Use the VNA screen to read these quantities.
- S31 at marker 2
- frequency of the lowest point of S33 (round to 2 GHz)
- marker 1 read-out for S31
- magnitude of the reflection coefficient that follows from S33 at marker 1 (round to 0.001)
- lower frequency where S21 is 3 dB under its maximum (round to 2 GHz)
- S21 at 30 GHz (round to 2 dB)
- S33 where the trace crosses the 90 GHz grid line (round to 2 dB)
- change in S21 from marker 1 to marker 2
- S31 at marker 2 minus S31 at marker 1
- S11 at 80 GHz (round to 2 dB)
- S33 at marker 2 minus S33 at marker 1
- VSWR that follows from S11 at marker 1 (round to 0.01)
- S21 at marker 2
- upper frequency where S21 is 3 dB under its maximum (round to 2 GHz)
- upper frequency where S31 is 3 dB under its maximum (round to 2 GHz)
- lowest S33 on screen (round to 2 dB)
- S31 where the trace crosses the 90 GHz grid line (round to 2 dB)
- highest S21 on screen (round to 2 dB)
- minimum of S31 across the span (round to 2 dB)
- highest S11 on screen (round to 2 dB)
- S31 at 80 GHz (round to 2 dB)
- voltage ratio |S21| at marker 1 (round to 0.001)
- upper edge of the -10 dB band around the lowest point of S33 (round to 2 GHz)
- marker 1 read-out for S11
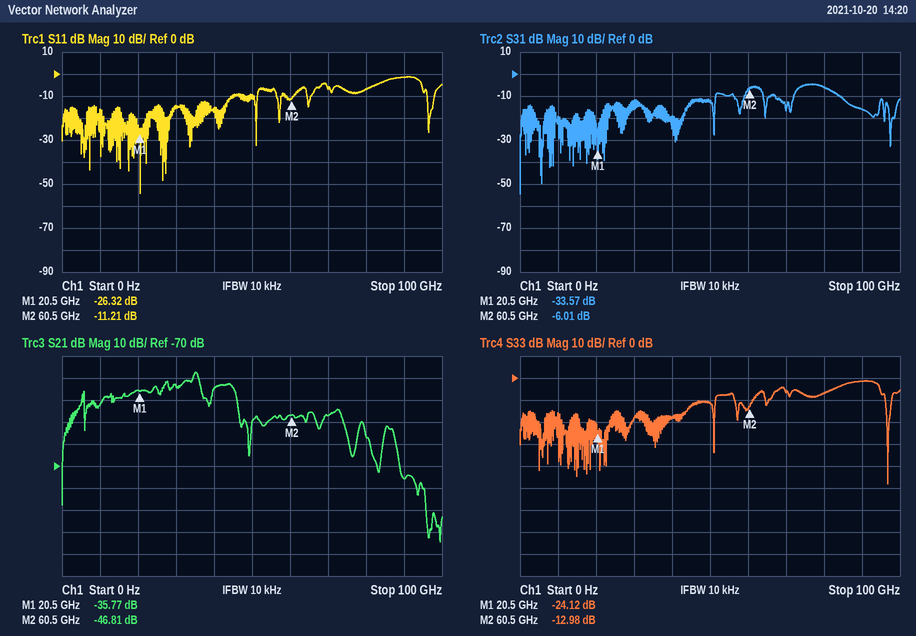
-6.01 dB
96 GHz
-33.57 dB
0.062
34 GHz
-34 dB
-2 dB
-11.04 dB
27.56 dB
-6 dB
11.14 dB
1.10
-46.81 dB
36 GHz
82 GHz
-48 dB
-16 dB
-28 dB
-54 dB
-2 dB
-6 dB
0.016
98 GHz
-26.32 dB
